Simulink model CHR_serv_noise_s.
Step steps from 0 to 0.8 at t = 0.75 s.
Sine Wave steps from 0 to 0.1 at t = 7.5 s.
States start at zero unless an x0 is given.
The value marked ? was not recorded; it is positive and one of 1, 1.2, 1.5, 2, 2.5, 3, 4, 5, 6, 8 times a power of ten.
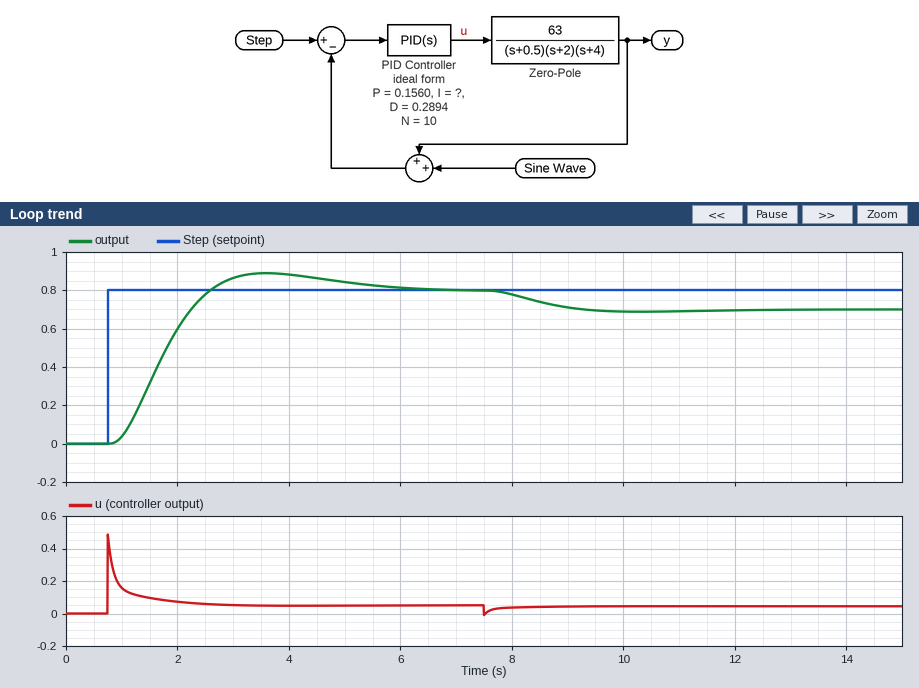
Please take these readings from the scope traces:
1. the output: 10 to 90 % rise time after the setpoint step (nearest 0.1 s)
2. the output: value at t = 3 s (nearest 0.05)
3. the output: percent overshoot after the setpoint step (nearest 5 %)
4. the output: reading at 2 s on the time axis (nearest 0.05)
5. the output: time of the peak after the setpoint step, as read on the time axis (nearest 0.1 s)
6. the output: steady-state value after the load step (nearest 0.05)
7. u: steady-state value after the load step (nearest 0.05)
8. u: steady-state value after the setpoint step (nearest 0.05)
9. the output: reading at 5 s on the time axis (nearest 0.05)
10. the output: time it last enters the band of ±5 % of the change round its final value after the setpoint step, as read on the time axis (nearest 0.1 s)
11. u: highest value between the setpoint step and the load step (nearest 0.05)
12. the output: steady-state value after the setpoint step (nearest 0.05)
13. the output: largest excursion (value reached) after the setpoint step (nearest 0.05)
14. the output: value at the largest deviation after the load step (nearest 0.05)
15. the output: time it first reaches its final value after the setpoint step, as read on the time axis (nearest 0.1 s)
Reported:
1.2 s
0.85
10 %
0.60
3.6 s
0.70
0.05
0.05
0.85
5.1 s
0.50
0.80
0.90
0.70
2.6 s
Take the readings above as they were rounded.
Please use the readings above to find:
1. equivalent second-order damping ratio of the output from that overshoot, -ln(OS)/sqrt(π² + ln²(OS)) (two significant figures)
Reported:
0.59
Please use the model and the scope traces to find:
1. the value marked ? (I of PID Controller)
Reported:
0.6
